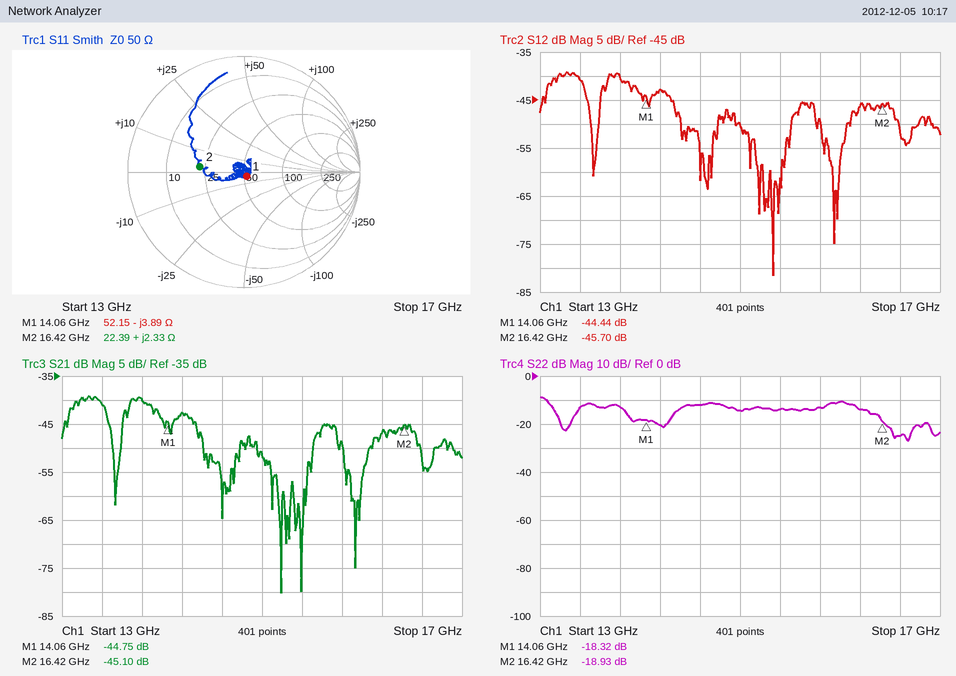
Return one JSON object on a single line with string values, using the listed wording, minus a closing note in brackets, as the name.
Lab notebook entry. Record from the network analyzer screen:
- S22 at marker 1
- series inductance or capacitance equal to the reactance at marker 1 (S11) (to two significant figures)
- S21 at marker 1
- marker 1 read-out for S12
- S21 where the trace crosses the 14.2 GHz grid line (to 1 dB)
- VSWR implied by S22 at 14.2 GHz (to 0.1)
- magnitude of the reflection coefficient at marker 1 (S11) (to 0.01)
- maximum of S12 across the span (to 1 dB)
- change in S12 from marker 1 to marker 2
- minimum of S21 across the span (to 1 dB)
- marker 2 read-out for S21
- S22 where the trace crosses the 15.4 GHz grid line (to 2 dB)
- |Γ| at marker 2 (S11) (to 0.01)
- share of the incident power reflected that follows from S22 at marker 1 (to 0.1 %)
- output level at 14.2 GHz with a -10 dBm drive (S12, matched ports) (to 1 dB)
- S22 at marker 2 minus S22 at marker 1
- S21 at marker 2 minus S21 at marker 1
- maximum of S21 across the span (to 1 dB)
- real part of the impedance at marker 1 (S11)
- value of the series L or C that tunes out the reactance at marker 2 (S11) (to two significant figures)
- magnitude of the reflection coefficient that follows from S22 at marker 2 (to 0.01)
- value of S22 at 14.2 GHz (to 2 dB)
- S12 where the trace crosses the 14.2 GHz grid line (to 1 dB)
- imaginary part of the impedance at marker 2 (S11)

{"S22 at marker 1": "-18.32 dB", "series inductance or capacitance equal to the reactance at marker 1 (S11)": "2.9 pF", "S21 at marker 1": "-44.75 dB", "marker 1 read-out for S12": "-44.44 dB", "S21 where the trace crosses the 14.2 GHz grid line": "-43 dB", "VSWR implied by S22 at 14.2 GHz": "1.2", "magnitude of the reflection coefficient at marker 1 (S11)": "0.04", "maximum of S12 across the span": "-39 dB", "change in S12 from marker 1 to marker 2": "-1.26 dB", "minimum of S21 across the span": "-80 dB", "marker 2 read-out for S21": "-45.10 dB", "S22 where the trace crosses the 15.4 GHz grid line": "-14 dB", "|Γ| at marker 2 (S11)": "0.38", "share of the incident power reflected that follows from S22 at marker 1": "1.5 %", "output level at 14.2 GHz with a -10 dBm drive (S12, matched ports)": "-53 dBm", "S22 at marker 2 minus S22 at marker 1": "-0.61 dB", "S21 at marker 2 minus S21 at marker 1": "-0.35 dB", "maximum of S21 across the span": "-39 dB", "real part of the impedance at marker 1": "52.15 Ω", "value of the series L or C that tunes out the reactance at marker 2 (S11)": "4.2 pF", "magnitude of the reflection coefficient that follows from S22 at marker 2": "0.11", "value of S22 at 14.2 GHz": "-20 dB", "S12 where the trace crosses the 14.2 GHz grid line": "-43 dB", "imaginary part of the impedance at marker 2": "+2.33 Ω"}
